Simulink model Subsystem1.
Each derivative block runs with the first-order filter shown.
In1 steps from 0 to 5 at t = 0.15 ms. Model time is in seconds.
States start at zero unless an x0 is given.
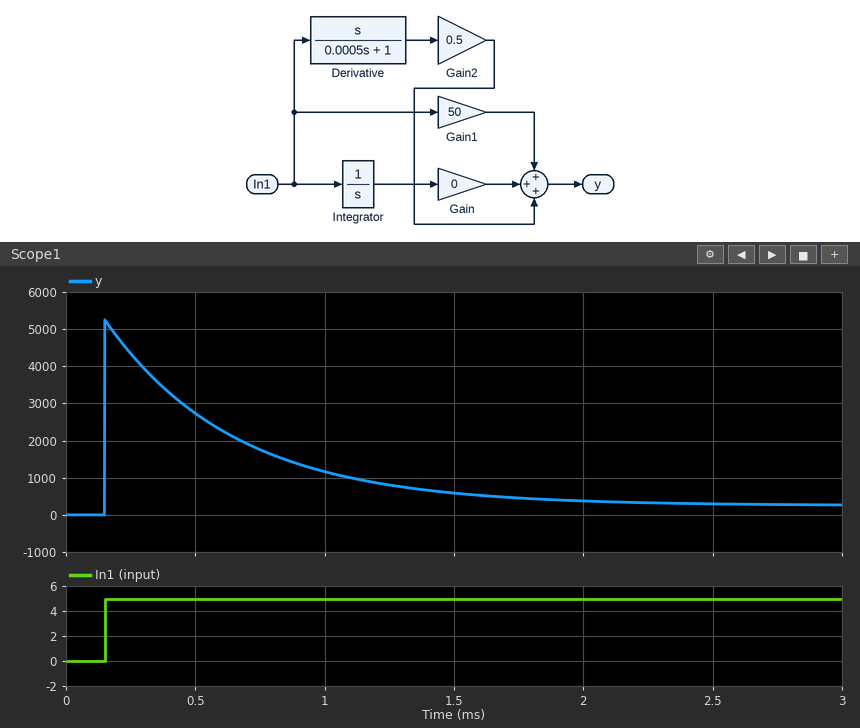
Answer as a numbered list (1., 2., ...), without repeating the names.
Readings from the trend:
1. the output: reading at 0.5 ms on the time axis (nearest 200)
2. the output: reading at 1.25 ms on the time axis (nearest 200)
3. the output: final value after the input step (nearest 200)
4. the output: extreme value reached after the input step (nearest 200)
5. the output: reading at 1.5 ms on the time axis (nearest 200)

1. 2800
2. 800
3. 200
4. 5200
5. 600
